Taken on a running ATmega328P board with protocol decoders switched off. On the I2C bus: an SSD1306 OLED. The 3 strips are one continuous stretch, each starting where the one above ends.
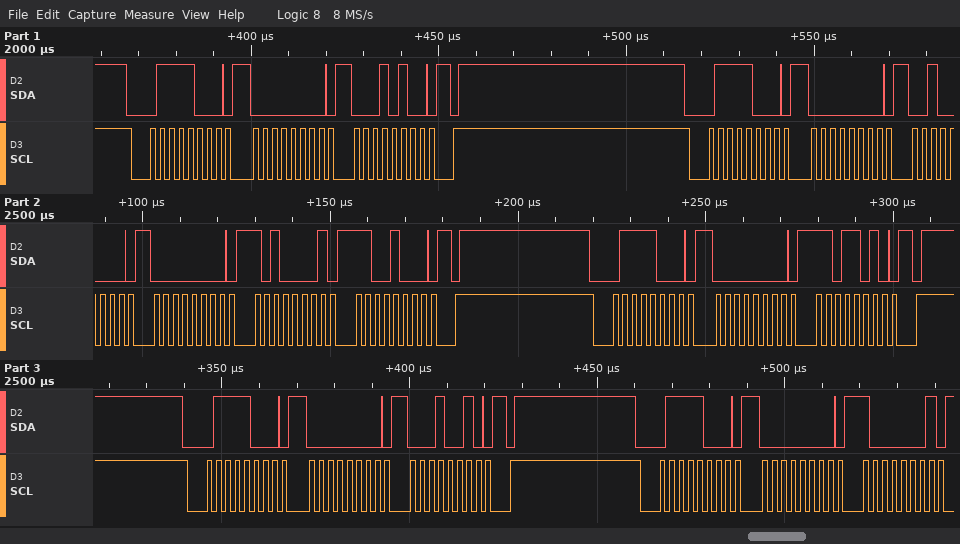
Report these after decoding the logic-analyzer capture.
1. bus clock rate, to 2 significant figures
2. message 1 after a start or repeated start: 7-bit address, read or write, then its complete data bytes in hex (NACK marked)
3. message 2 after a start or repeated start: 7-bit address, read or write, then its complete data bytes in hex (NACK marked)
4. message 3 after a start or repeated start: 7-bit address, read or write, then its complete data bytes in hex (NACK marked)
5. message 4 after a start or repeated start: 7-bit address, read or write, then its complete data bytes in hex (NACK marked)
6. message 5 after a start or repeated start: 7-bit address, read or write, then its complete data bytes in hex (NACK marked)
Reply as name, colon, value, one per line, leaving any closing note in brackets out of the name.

bus clock rate, to 2 significant figures: 400 kHz
message 1 after a start or repeated start: 7-bit address, read or write, then its complete data bytes in hex: 0x3C write: 00 14
message 2 after a start or repeated start: 7-bit address, read or write, then its complete data bytes in hex: 0x3C write: 00 20 00 A1 C8
message 3 after a start or repeated start: 7-bit address, read or write, then its complete data bytes in hex: 0x3C write: 00 DA
message 4 after a start or repeated start: 7-bit address, read or write, then its complete data bytes in hex: 0x3C write: 00 12
message 5 after a start or repeated start: 7-bit address, read or write, then its complete data bytes in hex: 0x3C write: 00 81
